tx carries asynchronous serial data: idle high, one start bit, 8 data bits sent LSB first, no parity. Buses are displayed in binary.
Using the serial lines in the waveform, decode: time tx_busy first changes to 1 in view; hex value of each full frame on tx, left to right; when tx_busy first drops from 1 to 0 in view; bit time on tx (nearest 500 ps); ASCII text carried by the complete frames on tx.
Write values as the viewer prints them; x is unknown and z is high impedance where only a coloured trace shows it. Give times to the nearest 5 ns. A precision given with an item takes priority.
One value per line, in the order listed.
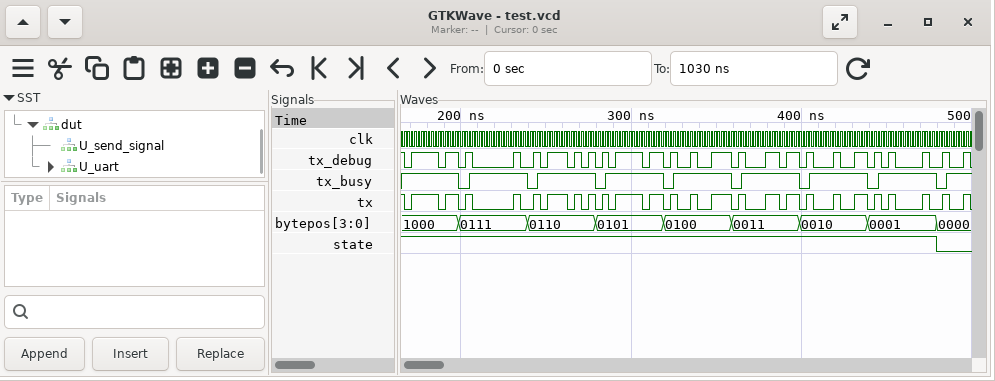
205 ns
6F, 20, 57, 6F, 72, 6C, 64, 21
200 ns
4000 ps
"o World!"
